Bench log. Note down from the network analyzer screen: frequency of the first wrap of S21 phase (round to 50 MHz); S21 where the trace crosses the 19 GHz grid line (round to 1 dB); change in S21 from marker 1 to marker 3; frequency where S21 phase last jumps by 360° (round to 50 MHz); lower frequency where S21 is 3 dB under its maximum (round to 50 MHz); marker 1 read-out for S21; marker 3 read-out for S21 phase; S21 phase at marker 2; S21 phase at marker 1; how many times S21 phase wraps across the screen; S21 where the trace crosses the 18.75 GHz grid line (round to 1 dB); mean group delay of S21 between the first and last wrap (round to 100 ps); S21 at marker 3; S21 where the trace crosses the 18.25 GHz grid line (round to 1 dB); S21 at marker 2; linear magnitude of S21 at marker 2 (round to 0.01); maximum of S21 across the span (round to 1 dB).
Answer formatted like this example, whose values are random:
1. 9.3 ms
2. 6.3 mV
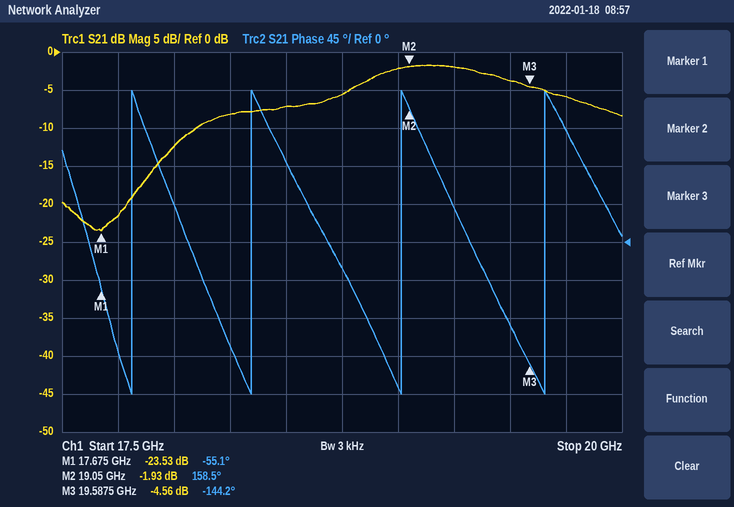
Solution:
1. 17.80 GHz
2. -2 dB
3. 18.97 dB
4. 19.65 GHz
5. 18.80 GHz
6. -23.53 dB
7. -144.2°
8. 158.5°
9. -55.1°
10. 4
11. -6 dB
12. 1.6 ns
13. -4.56 dB
14. -8 dB
15. -1.93 dB
16. 0.80
17. -2 dB
